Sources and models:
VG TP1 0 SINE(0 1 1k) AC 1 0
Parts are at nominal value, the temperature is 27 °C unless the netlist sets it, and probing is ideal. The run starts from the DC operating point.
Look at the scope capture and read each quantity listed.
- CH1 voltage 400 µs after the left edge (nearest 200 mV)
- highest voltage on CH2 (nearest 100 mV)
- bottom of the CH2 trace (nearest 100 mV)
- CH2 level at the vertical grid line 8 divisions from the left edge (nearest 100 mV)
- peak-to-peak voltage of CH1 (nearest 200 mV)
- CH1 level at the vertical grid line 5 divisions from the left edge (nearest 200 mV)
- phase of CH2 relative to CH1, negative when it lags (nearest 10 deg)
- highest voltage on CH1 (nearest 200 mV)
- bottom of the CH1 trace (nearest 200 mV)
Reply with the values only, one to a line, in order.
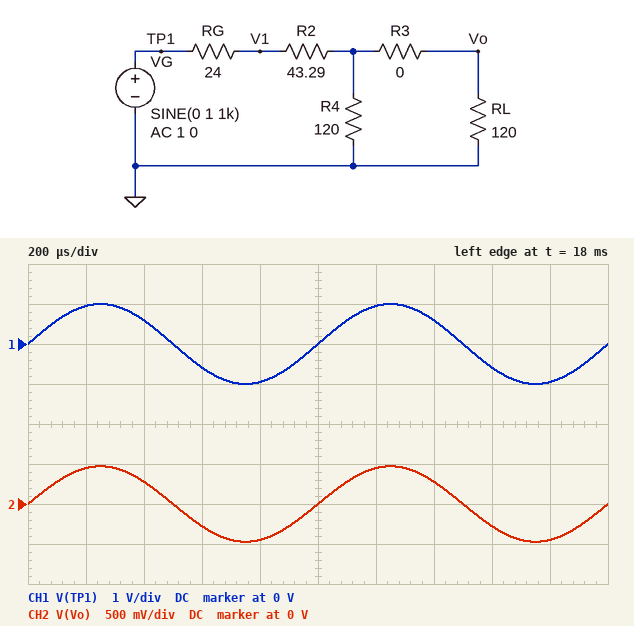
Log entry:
600 mV
500 mV
-500 mV
-300 mV
2.0 V
0 V
0 deg
1.0 V
-1.0 V
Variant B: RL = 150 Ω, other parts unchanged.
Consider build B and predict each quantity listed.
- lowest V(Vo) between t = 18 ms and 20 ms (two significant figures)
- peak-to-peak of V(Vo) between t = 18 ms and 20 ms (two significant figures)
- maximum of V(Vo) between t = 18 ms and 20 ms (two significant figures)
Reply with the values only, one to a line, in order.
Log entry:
-500 mV
990 mV
500 mV
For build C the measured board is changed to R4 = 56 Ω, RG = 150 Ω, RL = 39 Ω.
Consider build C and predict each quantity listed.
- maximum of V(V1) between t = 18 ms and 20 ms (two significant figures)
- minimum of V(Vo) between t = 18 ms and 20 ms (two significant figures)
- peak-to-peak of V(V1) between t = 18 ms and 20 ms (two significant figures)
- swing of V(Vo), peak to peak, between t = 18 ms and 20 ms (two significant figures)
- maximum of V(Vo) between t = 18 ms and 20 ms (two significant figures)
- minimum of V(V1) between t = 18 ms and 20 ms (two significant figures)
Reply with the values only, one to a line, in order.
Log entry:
310 mV
-110 mV
610 mV
210 mV
110 mV
-310 mV
